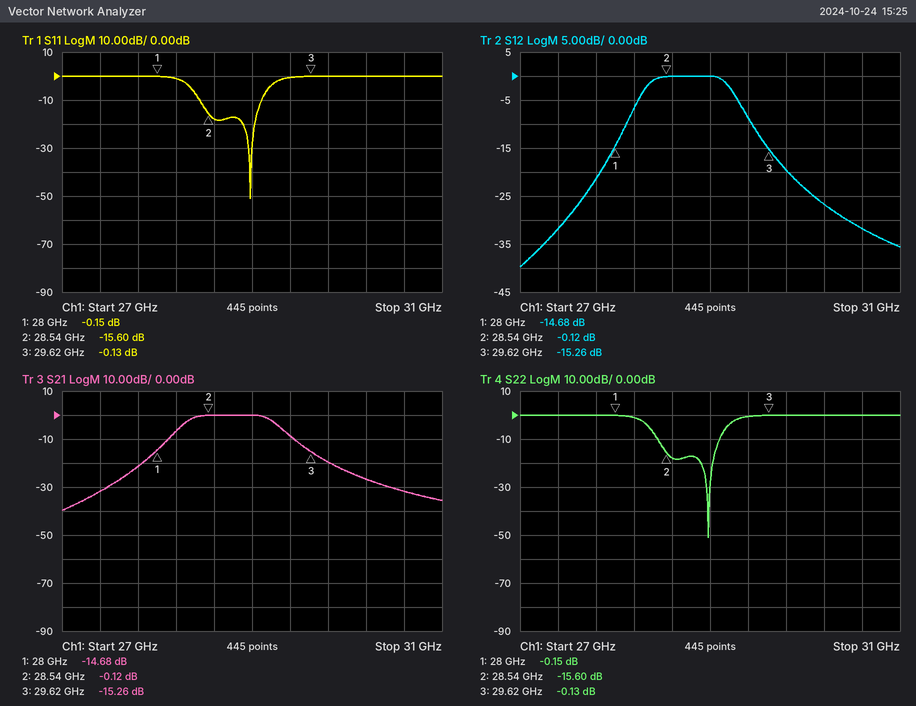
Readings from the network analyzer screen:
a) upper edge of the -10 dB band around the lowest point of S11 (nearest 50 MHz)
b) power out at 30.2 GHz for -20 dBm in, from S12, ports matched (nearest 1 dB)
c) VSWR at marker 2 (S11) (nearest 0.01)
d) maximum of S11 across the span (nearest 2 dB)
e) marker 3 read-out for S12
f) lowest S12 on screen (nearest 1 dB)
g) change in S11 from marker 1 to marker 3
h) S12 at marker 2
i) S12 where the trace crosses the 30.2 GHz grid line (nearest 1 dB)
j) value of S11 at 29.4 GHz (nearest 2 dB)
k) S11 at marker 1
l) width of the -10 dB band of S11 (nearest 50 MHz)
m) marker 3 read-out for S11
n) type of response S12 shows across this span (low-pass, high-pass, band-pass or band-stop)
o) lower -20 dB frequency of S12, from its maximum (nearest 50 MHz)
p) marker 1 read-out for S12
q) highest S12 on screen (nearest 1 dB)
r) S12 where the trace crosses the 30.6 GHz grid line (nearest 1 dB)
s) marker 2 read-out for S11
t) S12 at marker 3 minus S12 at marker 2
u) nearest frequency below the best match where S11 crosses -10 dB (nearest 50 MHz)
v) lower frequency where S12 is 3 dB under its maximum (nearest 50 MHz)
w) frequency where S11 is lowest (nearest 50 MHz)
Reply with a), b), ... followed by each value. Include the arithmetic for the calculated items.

a) 29.10 GHz
b) -20 dBm + (-27 dB) = -47 dBm
c) (1 + 0.1660)/(1 − 0.1660) ≈ 1.40
d) 0 dB
e) -15.26 dB
f) -40 dB
g) -0.13 − (-0.15) = 0.02 dB
h) -0.12 dB
i) -27 dB
j) 0 dB
k) -0.15 dB
l) 29.10 GHz − 28.45 GHz = 650 MHz
m) -0.13 dB
n) band-pass
o) 27.85 GHz
p) -14.68 dB
q) 0 dB
r) -32 dB
s) -15.60 dB
t) -15.26 − (-0.12) = -15.14 dB
u) 28.45 GHz
v) 28.30 GHz
w) 29.00 GHz
